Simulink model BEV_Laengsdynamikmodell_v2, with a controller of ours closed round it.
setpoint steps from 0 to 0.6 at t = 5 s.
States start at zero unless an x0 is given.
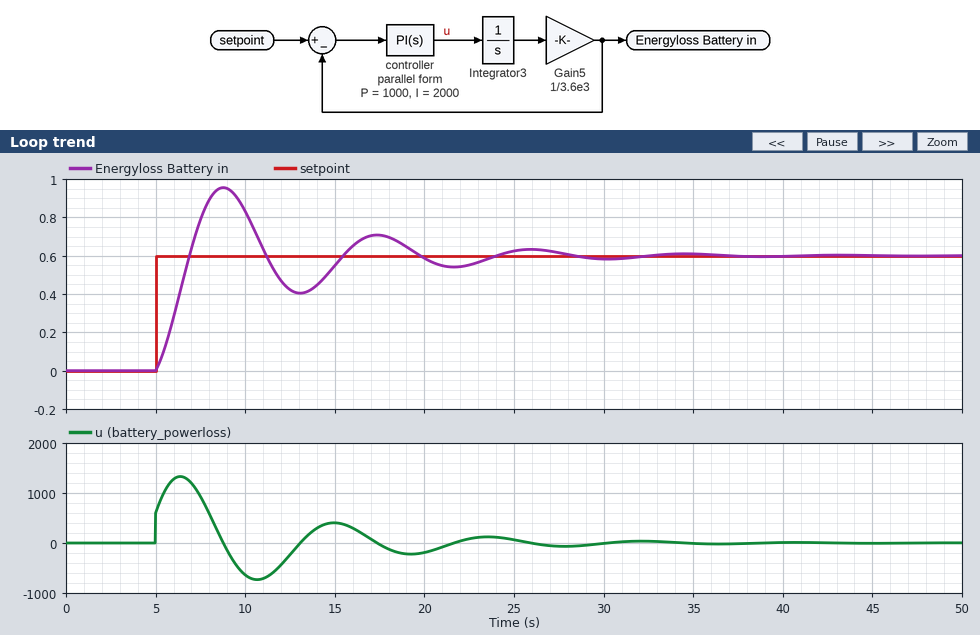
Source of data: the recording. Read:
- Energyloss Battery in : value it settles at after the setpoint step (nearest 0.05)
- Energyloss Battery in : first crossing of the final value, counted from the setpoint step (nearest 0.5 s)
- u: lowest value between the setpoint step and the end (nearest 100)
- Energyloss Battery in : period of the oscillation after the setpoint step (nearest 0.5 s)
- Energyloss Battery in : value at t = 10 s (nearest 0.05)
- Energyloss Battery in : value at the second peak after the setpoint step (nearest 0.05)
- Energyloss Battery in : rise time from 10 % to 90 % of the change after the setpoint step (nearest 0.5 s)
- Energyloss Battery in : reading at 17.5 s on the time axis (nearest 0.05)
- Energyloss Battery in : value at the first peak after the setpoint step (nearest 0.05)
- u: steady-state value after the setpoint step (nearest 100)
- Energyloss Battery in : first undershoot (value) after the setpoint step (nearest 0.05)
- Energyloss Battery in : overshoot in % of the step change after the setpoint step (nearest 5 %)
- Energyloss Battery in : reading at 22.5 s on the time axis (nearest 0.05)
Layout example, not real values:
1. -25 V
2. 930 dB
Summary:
1. 0.60
2. 2.0 s
3. -700
4. 8.5 s
5. 0.85
6. 0.70
7. 1.5 s
8. 0.70
9. 0.95
10. 0
11. 0.40
12. 60 %
13. 0.55
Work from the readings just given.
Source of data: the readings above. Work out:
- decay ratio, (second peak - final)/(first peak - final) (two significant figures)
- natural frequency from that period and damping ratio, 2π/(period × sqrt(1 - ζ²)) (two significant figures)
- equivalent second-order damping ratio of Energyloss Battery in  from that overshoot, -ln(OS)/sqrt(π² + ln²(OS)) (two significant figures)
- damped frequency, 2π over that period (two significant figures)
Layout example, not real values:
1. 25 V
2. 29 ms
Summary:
1. 0.29
2. 0.75 rad/s
3. 0.16
4. 0.74 rad/s
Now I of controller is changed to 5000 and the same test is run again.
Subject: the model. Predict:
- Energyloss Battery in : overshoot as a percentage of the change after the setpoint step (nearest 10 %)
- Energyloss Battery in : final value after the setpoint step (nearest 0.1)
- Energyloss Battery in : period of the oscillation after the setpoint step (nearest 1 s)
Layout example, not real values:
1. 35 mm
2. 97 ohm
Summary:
1. 70 %
2. 0.6
3. 5 s
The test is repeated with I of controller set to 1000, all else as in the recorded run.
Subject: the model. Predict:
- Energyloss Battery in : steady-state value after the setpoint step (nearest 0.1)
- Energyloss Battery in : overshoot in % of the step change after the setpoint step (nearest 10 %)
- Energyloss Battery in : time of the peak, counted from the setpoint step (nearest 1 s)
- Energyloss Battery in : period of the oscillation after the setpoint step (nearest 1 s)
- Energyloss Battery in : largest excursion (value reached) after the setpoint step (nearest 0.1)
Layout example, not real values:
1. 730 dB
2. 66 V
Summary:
1. 0.6
2. 50 %
3. 5 s
4. 12 s
5. 0.9
